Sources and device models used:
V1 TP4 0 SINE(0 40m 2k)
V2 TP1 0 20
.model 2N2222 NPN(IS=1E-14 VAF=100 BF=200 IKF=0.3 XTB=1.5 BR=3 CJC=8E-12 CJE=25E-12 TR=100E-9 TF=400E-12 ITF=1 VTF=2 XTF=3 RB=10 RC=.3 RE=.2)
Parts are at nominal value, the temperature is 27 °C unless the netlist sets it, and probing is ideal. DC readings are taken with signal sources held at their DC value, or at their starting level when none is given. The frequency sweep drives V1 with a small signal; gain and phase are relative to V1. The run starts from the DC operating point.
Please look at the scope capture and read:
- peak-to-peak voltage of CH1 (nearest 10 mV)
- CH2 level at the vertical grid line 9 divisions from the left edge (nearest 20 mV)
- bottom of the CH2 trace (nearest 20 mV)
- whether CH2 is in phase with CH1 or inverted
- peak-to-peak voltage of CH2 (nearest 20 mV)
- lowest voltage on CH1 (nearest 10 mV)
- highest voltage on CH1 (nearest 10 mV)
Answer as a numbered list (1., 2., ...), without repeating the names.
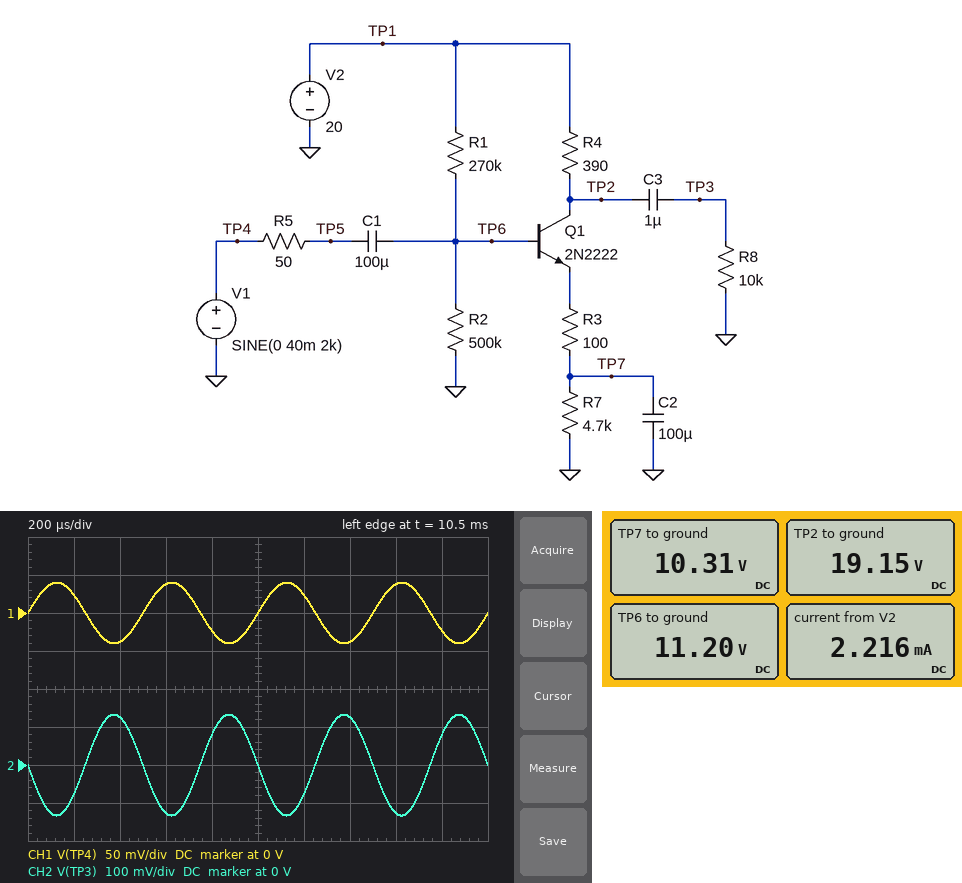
1. 80 mV
2. 80 mV
3. -140 mV
4. inverted
5. 260 mV
6. -40 mV
7. 40 mV
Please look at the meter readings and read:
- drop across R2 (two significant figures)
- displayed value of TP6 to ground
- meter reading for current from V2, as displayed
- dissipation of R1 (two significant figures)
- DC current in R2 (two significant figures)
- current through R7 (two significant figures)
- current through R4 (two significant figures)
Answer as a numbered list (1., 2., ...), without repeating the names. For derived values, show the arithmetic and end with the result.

1. 11.2 V = 11 V
2. 11.20 V
3. 2.216 mA
4. (20 V - 11.2 V)^2 / 270 kΩ = 290 µW
5. (11.2 V) / 500 kΩ = 22 µA
6. (10.31 V) / 4.7 kΩ = 2.2 mA
7. (20 V - 19.15 V) / 390 Ω = 2.2 mA
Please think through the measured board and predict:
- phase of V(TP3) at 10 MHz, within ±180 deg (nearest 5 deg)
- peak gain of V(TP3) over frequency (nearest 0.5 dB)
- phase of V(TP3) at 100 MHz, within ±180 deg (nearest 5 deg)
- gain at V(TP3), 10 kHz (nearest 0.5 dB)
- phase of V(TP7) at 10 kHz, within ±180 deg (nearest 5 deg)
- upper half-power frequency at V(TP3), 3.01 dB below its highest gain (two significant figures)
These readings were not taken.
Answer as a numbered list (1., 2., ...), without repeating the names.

1. 165 deg
2. 10.5 dB
3. 85 deg
4. 10.5 dB
5. -90 deg
6. 58 MHz
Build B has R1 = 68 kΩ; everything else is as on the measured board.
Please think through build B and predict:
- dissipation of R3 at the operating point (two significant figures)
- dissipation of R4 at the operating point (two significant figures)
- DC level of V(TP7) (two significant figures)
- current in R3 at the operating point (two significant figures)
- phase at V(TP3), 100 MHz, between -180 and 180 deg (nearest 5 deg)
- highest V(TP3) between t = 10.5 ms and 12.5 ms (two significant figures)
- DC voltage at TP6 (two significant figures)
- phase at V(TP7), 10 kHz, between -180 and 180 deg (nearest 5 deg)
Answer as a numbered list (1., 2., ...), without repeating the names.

1. 1.1 mW
2. 4.3 mW
3. 16 V
4. 3.3 mA
5. 75 deg
6. 140 mV
7. 17 V
8. -90 deg
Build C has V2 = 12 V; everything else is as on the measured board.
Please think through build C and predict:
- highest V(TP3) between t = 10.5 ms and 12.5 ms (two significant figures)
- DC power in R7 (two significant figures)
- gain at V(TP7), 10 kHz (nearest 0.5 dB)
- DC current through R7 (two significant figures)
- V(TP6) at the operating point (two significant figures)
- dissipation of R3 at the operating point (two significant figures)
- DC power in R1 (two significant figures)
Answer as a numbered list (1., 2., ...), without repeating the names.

1. 120 mV
2. 7.5 mW
3. -57.5 dB
4. 1.3 mA
5. 6.7 V
6. 160 µW
7. 100 µW
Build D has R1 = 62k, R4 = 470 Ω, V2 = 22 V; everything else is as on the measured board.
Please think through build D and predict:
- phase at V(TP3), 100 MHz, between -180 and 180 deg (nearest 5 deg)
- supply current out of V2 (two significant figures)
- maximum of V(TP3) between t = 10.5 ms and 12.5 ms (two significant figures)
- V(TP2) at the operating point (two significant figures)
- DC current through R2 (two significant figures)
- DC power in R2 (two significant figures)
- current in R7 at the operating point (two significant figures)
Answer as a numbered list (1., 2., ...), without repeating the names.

1. 70 deg
2. 3.8 mA
3. 170 mV
4. 20 V
5. 37 µA
6. 690 µW
7. 3.7 mA
